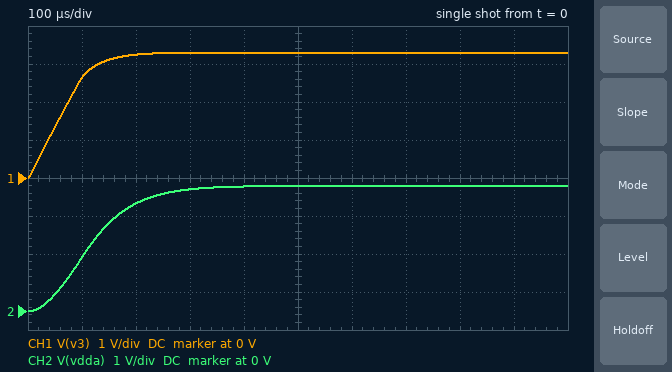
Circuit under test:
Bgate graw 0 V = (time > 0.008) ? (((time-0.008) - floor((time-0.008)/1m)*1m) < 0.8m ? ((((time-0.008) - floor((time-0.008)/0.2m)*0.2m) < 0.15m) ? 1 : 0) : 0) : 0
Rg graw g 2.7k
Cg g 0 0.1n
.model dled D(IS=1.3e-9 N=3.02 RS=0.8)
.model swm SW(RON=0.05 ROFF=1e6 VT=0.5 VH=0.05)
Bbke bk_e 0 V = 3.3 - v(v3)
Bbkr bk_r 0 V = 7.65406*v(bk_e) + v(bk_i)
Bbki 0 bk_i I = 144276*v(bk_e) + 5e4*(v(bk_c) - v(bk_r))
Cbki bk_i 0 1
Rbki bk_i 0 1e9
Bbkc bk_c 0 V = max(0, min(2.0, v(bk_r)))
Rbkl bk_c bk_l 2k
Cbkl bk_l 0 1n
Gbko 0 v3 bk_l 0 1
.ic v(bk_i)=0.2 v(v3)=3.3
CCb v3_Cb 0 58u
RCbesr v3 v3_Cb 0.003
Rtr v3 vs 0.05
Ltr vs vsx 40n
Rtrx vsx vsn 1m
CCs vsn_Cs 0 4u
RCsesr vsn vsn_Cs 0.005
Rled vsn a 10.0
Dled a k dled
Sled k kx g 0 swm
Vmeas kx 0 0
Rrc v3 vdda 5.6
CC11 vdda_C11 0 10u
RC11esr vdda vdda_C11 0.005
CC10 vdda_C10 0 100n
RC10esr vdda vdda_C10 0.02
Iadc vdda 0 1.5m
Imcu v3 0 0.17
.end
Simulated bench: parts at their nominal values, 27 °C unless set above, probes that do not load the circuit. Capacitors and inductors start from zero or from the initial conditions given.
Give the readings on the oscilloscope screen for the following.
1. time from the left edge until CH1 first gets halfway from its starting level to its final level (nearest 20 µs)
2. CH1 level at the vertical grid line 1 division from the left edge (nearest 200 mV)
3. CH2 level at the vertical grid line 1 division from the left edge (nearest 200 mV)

60 µs
2.6 V
1.4 V
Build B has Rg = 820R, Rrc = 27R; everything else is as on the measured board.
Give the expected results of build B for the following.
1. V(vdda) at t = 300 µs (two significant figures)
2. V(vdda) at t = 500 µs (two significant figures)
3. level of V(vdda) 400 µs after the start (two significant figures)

1.9 V
2.6 V
2.3 V
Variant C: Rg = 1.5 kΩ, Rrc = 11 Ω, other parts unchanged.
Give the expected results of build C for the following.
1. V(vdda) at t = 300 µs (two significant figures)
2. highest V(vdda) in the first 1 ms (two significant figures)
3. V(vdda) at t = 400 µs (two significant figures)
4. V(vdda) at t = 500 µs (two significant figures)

2.8 V
3.3 V
3.1 V
3.2 V
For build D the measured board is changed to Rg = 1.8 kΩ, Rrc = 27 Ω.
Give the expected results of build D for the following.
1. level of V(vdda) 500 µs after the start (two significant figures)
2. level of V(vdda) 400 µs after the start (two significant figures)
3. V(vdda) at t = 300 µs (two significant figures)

2.6 V
2.3 V
1.9 V
